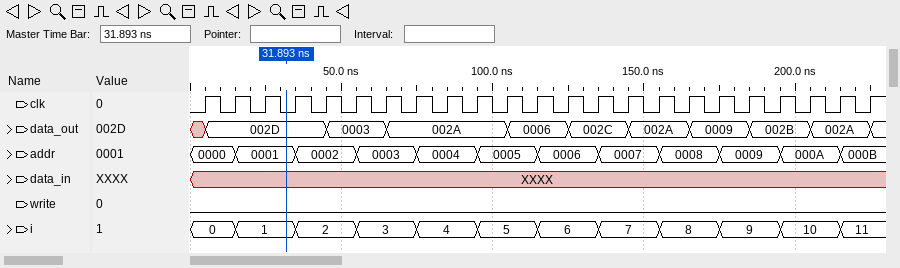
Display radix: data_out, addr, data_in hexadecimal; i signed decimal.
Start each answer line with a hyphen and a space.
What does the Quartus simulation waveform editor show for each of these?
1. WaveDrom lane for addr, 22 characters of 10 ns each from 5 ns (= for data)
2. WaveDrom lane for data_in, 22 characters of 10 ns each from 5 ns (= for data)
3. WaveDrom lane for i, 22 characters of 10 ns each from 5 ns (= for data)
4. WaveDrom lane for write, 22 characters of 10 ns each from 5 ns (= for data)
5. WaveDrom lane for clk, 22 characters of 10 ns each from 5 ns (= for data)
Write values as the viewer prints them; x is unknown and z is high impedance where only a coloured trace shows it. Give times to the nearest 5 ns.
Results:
- {name: 'addr', wave: '==.=.=.=.=.=.=.=.=.=.=', data: '0000 0001 0002 0003 0004 0005 0006 0007 0008 0009 000A 000B'}
- {name: 'data_in', wave: 'x.....................'}
- {name: 'i', wave: '==.=.=.=.=.=.=.=.=.=.=', data: '0 1 2 3 4 5 6 7 8 9 10 11'}
- {name: 'write', wave: '0.....................'}
- {name: 'clk', wave: 'p.....................'}
